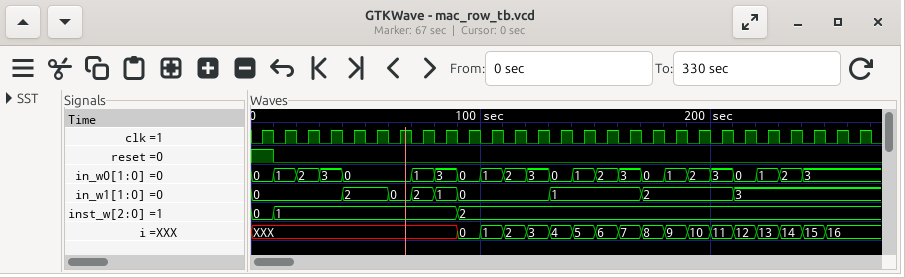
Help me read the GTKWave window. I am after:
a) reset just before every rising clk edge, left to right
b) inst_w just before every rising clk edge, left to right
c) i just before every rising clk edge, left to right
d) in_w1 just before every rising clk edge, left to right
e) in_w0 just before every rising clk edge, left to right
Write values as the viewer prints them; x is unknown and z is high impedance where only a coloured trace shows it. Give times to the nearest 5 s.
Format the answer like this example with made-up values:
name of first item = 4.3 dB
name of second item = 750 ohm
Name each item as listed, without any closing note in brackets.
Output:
reset just before every rising clk edge, left to right = 1 0 0 0 0 0 0 0 0 0 0 0 0 0 0 0 0 0 0 0 0 0 0 0 0 0 0
inst_w just before every rising clk edge, left to right = 0, 1, 1, 1, 1, 1, 1, 1, 1, 2, 2, 2, 2, 2, 2, 2, 2, 2, 2, 2, 2, 2, 2, 2, 2, 2, 2
i just before every rising clk edge, left to right = XXX, XXX, XXX, XXX, XXX, XXX, XXX, XXX, XXX, 0, 1, 2, 3, 4, 5, 6, 7, 8, 9, 10, 11, 12, 13, 14, 15, 16, 16
in_w1 just before every rising clk edge, left to right = 0, 0, 0, 0, 2, 2, 0, 2, 1, 0, 0, 0, 0, 1, 1, 1, 1, 2, 2, 2, 2, 3, 3, 3, 3, 3, 3
in_w0 just before every rising clk edge, left to right = 0, 1, 2, 3, 0, 0, 0, 1, 3, 0, 1, 2, 3, 0, 1, 2, 3, 0, 1, 2, 3, 0, 1, 2, 3, 3, 3
